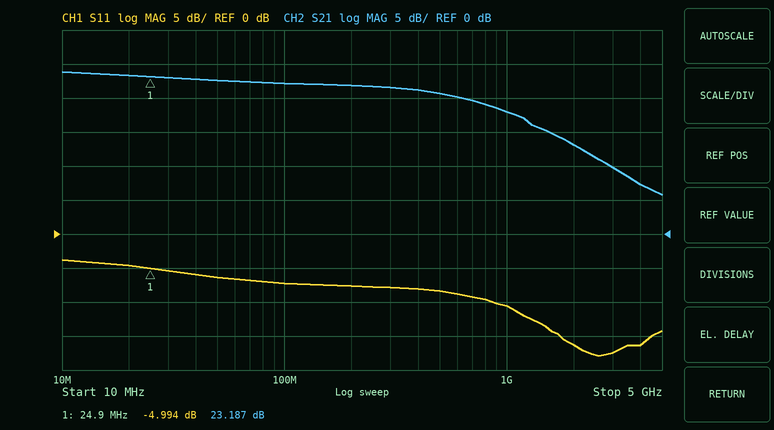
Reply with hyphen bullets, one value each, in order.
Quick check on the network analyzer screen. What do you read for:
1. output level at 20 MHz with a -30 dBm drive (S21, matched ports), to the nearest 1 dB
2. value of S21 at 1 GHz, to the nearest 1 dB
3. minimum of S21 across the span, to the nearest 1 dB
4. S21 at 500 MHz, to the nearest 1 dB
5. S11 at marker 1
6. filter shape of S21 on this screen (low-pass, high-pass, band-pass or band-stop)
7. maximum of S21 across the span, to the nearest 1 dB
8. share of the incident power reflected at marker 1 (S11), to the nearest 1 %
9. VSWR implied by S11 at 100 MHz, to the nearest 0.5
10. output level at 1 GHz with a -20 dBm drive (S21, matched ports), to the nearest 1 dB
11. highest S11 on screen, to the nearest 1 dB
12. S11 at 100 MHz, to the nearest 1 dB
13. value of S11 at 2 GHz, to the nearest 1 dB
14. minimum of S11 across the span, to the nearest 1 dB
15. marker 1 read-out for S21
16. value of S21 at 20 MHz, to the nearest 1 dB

- -7 dBm
- 18 dB
- 6 dB
- 21 dB
- -4.994 dB
- low-pass
- 24 dB
- 32 %
- 2.5
- -2 dBm
- -4 dB
- -7 dB
- -16 dB
- -18 dB
- 23.187 dB
- 23 dB
